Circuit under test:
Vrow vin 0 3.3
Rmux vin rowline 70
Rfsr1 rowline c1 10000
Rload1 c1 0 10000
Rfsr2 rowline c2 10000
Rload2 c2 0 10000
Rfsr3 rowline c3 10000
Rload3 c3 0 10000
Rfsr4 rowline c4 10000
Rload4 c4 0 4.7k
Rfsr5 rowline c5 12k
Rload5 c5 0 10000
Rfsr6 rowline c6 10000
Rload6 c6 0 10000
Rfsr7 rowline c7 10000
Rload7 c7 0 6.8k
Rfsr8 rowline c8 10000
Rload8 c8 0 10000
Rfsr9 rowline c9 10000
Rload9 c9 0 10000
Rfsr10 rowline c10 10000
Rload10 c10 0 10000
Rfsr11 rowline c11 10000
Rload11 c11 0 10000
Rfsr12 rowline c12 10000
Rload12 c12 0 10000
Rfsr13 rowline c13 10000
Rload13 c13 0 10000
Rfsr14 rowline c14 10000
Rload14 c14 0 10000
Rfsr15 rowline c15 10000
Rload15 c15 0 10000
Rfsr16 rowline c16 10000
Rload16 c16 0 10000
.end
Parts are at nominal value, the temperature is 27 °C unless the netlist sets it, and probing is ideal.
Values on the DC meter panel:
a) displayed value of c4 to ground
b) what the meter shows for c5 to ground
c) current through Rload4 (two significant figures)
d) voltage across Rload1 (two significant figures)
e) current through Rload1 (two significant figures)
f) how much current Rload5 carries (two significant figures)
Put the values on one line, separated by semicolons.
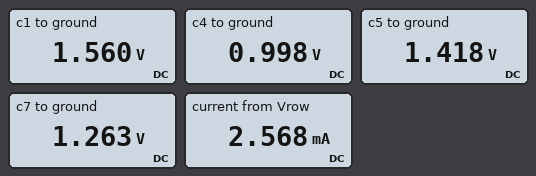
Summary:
0.998 V; 1.418 V; 210 µA; 1.6 V; 160 µA; 140 µA
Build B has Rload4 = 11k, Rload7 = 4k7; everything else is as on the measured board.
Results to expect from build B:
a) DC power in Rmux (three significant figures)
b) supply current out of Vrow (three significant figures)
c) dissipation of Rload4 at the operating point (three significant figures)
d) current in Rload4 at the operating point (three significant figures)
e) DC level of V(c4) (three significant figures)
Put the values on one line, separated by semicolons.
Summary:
449 µW; 2.53 mA; 243 µW; 149 µA; 1.64 V
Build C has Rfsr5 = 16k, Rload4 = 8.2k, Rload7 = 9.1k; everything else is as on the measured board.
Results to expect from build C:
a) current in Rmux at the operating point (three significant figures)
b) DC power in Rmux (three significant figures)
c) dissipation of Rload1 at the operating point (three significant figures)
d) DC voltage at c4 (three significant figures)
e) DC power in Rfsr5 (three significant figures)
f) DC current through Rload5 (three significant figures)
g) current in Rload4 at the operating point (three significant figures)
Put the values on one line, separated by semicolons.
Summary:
2.49 mA; 433 µW; 244 µW; 1.41 V; 231 µW; 120 µA; 172 µA
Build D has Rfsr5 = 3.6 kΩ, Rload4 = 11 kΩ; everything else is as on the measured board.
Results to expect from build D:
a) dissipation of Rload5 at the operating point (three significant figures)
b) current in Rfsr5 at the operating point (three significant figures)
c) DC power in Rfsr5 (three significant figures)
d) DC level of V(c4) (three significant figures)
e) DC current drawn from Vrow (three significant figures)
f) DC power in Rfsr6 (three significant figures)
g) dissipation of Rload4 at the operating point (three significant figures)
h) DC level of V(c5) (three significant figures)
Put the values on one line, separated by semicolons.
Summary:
526 µW; 229 µA; 189 µW; 1.63 V; 2.59 mA; 243 µW; 243 µW; 2.29 V
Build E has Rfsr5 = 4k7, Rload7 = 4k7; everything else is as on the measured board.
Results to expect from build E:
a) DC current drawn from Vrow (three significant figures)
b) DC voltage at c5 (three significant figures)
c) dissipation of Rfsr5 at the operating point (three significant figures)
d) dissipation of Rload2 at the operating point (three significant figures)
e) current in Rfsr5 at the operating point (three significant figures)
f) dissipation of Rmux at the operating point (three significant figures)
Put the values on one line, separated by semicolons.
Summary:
2.66 mA; 2.12 V; 211 µW; 242 µW; 212 µA; 495 µW
